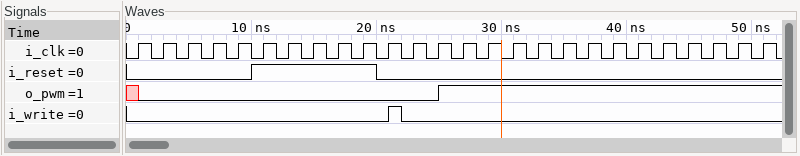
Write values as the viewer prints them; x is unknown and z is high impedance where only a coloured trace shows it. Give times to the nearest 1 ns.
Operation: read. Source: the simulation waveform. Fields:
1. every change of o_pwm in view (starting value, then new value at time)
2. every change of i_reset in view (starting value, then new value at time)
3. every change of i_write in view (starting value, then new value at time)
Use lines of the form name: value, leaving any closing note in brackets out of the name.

every change of o_pwm in view: x, 0 at 1 ns, 1 at 25 ns
every change of i_reset in view: 0, 1 at 10 ns, 0 at 20 ns
every change of i_write in view: 0, 1 at 21 ns, 0 at 22 ns
